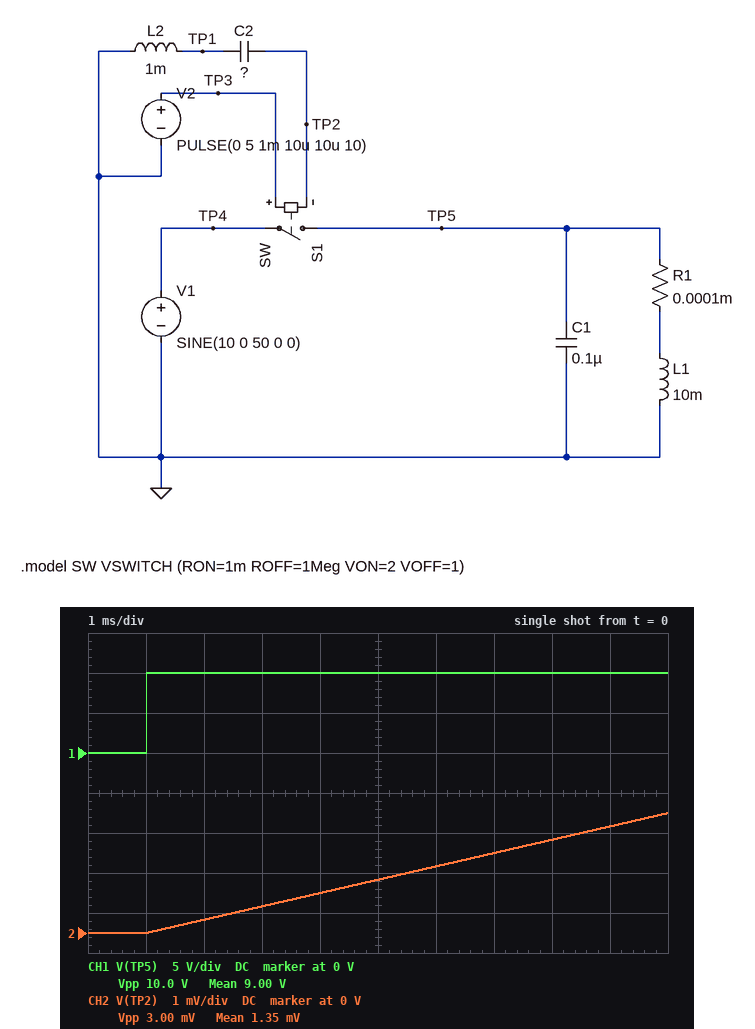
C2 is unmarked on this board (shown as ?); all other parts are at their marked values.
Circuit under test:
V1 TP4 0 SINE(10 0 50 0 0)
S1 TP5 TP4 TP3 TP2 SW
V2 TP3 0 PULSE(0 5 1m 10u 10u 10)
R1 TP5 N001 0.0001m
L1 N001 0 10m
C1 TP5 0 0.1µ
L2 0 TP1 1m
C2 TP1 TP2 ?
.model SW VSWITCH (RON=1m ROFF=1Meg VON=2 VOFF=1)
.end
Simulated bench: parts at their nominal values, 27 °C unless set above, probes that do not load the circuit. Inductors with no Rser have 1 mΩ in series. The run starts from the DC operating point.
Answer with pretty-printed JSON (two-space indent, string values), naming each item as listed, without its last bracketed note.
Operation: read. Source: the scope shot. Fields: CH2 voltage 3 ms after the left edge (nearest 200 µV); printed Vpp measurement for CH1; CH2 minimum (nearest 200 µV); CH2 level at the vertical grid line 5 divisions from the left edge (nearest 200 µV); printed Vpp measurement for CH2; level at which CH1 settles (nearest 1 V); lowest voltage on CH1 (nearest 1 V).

{
  "CH2 voltage 3 ms after the left edge": "600 µV",
  "printed Vpp measurement for CH1": "10.0 V",
  "CH2 minimum": "0 V",
  "CH2 level at the vertical grid line 5 divisions from the left edge": "1.4 mV",
  "printed Vpp measurement for CH2": "3.00 mV",
  "level at which CH1 settles": "10 V",
  "lowest voltage on CH1": "0 V"
}
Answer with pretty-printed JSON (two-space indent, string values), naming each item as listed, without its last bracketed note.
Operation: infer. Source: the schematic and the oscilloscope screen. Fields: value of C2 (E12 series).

{
  "value of C2": "15 pF"
}
